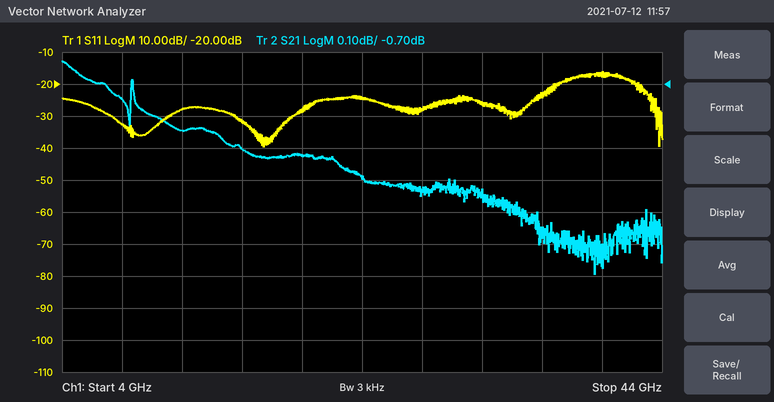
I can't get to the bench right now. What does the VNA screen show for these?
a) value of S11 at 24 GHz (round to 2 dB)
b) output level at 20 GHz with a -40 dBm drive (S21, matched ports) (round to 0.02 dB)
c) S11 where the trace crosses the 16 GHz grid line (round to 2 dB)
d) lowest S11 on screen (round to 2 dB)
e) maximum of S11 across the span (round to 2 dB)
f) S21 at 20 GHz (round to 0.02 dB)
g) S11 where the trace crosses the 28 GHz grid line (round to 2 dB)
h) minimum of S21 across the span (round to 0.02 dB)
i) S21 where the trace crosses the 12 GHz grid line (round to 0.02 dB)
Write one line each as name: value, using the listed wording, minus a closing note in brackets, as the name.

value of S11 at 24 GHz: -24 dB
output level at 20 GHz with a -40 dBm drive (S21, matched ports): -40.92 dBm
S11 where the trace crosses the 16 GHz grid line: -32 dB
lowest S11 on screen: -40 dB
maximum of S11 across the span: -16 dB
S21 at 20 GHz: -0.92 dB
S11 where the trace crosses the 28 GHz grid line: -28 dB
minimum of S21 across the span: -1.30 dB
S21 where the trace crosses the 12 GHz grid line: -0.84 dB
